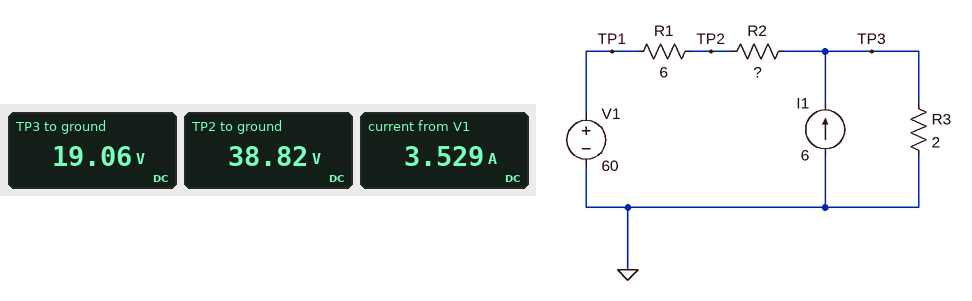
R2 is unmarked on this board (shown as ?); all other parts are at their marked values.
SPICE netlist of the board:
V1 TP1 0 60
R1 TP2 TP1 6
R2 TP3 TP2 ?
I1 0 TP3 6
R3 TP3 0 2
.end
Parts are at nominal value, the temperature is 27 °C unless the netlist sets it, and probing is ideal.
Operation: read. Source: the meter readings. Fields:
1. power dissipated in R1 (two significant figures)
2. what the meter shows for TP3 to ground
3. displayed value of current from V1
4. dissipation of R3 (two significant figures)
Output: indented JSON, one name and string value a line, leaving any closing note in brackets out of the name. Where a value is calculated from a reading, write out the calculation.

{
  "power dissipated in R1": "(60 V - 38.82 V)^2 / 6 Ω = 75 W",
  "what the meter shows for TP3 to ground": "19.06 V",
  "displayed value of current from V1": "3.529 A",
  "dissipation of R3": "(19.06 V)^2 / 2 Ω = 180 W"
}
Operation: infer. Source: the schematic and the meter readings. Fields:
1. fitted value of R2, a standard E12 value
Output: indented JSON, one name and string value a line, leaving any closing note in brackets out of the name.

{
  "fitted value of R2, a standard E12 value": "5.6 Ω"
}
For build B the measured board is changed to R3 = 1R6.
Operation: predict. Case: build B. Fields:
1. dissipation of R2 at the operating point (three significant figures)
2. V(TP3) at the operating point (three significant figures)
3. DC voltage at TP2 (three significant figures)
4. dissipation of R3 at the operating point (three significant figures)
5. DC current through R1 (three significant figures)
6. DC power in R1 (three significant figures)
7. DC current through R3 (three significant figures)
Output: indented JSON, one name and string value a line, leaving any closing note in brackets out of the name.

{
  "dissipation of R2 at the operating point": "81.6 W",
  "V(TP3) at the operating point": "15.7 V",
  "DC voltage at TP2": "37.1 V",
  "dissipation of R3 at the operating point": "154 W",
  "DC current through R1": "3.82 A",
  "DC power in R1": "87.5 W",
  "DC current through R3": "9.82 A"
}
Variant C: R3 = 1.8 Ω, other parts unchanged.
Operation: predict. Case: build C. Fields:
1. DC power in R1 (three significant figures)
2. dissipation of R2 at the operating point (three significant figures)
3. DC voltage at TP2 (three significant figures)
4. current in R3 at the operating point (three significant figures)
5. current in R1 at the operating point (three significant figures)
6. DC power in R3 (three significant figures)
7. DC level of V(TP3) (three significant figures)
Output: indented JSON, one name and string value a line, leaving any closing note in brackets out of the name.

{
  "DC power in R1": "80.9 W",
  "dissipation of R2 at the operating point": "75.5 W",
  "DC voltage at TP2": "38.0 V",
  "current in R3 at the operating point": "9.67 A",
  "current in R1 at the operating point": "3.67 A",
  "DC power in R3": "168 W",
  "DC level of V(TP3)": "17.4 V"
}
